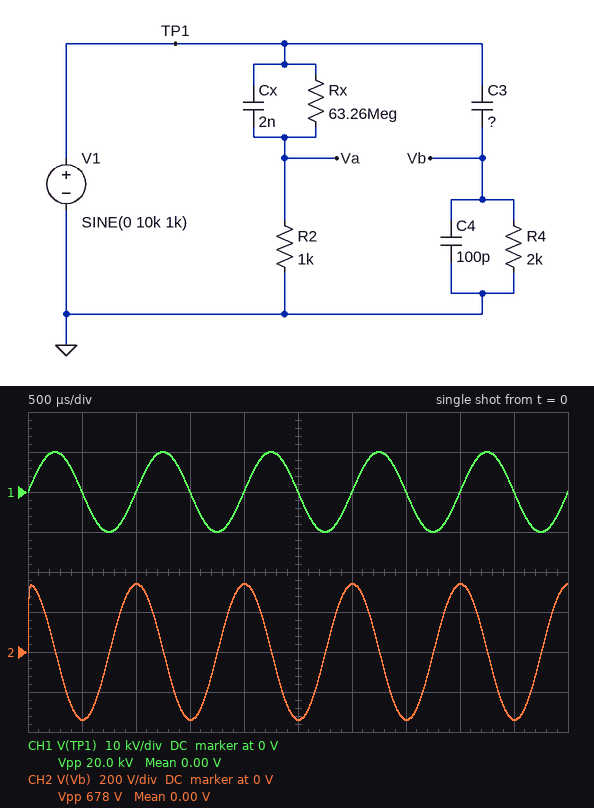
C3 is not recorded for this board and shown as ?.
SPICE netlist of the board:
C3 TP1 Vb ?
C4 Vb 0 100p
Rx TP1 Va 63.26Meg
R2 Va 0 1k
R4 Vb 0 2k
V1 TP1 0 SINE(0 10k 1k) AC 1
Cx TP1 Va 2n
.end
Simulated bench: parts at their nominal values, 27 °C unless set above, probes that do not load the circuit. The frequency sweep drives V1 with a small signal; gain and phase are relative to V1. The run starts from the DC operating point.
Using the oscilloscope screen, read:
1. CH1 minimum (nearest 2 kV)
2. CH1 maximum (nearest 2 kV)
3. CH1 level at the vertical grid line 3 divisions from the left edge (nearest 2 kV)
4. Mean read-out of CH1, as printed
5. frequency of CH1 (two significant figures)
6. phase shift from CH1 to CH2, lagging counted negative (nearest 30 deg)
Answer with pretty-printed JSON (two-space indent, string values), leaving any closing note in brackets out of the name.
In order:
{
  "CH1 minimum": "-10 kV",
  "CH1 maximum": "10 kV",
  "CH1 level at the vertical grid line 3 divisions from the left edge": "0 V",
  "Mean read-out of CH1, as printed": "0.00 V",
  "frequency of CH1": "1.0 kHz",
  "phase shift from CH1 to CH2, lagging counted negative": "90 deg"
}
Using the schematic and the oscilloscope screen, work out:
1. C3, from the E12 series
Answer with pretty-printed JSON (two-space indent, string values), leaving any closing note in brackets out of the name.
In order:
{
  "C3, from the E12 series": "2.7 nF"
}
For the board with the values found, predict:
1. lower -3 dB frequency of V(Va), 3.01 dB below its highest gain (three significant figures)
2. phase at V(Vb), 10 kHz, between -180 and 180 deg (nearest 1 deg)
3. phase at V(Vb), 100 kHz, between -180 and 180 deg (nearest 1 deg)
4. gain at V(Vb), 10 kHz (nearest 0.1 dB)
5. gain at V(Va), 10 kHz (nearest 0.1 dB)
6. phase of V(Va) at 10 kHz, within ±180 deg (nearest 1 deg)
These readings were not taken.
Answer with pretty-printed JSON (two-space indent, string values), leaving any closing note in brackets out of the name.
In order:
{
  "lower -3 dB frequency of V(Va), 3.01 dB below its highest gain": "79.6 kHz",
  "phase at V(Vb), 10 kHz, between -180 and 180 deg": "71 deg",
  "phase at V(Vb), 100 kHz, between -180 and 180 deg": "16 deg",
  "gain at V(Vb), 10 kHz": "-9.9 dB",
  "gain at V(Va), 10 kHz": "-18.1 dB",
  "phase of V(Va) at 10 kHz, within ±180 deg": "83 deg"
}
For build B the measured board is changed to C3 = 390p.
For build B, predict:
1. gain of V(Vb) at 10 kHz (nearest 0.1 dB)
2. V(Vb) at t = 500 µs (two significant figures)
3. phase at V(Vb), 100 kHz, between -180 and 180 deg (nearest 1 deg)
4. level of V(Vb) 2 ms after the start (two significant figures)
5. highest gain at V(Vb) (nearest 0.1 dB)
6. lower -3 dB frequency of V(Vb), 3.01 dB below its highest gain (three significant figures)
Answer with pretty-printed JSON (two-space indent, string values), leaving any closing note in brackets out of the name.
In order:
{
  "gain of V(Vb) at 10 kHz": "-26.2 dB",
  "V(Vb) at t = 500 µs": "-49 V",
  "phase at V(Vb), 100 kHz, between -180 and 180 deg": "58 deg",
  "level of V(Vb) 2 ms after the start": "49 V",
  "highest gain at V(Vb)": "-2.0 dB",
  "lower -3 dB frequency of V(Vb), 3.01 dB below its highest gain": "162 kHz"
}
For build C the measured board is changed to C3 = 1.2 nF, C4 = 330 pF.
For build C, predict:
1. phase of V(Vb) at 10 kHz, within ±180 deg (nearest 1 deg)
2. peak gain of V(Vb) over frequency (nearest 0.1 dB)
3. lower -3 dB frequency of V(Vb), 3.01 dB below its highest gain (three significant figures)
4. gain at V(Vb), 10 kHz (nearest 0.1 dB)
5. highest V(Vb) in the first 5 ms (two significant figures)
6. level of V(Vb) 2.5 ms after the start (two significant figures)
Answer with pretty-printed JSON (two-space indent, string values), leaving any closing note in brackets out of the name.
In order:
{
  "phase of V(Vb) at 10 kHz, within ±180 deg": "79 deg",
  "peak gain of V(Vb) over frequency": "-2.1 dB",
  "lower -3 dB frequency of V(Vb), 3.01 dB below its highest gain": "52.0 kHz",
  "gain at V(Vb), 10 kHz": "-16.6 dB",
  "highest V(Vb) in the first 5 ms": "150 V",
  "level of V(Vb) 2.5 ms after the start": "-150 V"
}
